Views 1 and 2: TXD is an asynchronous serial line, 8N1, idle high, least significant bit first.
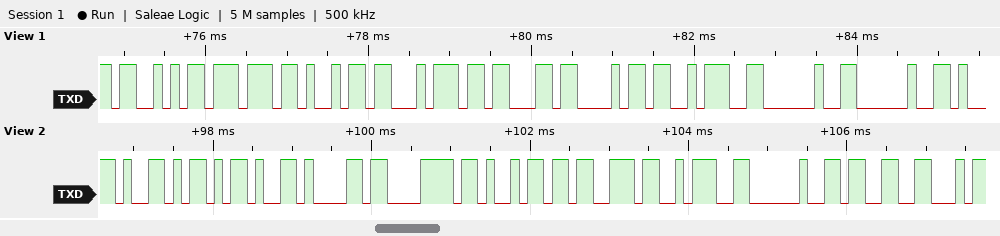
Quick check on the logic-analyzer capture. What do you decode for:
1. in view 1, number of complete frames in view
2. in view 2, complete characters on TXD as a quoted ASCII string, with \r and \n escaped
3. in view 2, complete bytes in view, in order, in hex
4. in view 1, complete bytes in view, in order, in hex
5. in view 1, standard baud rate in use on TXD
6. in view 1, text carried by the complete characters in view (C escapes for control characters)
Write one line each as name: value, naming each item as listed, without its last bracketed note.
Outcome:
in view 1, number of complete frames in view: 9
in view 2, complete characters on TXD as a quoted ASCII string, with \r and \n escaped: "Y-axis: 3"
in view 2, complete bytes in view, in order, in hex: 59 2D 61 78 69 73 3A 20 33
in view 1, complete bytes in view, in order, in hex: 53 77 69 74 63 68 3A 20 20
in view 1, standard baud rate in use on TXD: 9600 baud
in view 1, text carried by the complete characters in view: "Switch:  "
